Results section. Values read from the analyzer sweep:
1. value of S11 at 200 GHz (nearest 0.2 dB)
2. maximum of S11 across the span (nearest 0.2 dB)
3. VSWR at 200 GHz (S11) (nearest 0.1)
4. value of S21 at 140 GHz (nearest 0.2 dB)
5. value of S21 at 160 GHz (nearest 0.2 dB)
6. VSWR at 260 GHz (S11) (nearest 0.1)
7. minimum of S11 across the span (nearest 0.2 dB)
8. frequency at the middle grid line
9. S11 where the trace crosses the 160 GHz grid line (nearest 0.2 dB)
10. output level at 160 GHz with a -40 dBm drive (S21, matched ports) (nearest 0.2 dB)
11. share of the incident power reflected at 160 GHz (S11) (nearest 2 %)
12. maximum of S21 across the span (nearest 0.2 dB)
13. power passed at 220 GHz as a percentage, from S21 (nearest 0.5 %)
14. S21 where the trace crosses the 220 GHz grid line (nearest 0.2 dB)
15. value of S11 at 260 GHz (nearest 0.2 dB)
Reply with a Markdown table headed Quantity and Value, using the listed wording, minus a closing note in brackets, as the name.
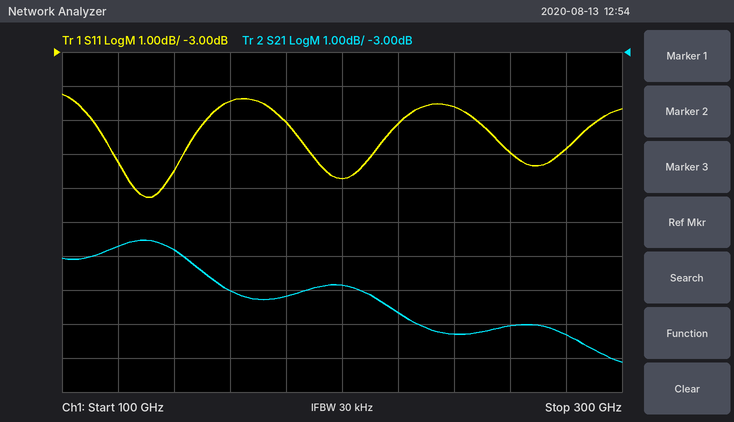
| Quantity | Value |
|---|---|
| value of S11 at 200 GHz | -6.8 dB |
| maximum of S11 across the span | -4.2 dB |
| VSWR at 200 GHz (S11) | 2.7 |
| value of S21 at 140 GHz | -8.8 dB |
| value of S21 at 160 GHz | -10.0 dB |
| VSWR at 260 GHz (S11) | 3.0 |
| minimum of S11 across the span | -7.2 dB |
| frequency at the middle grid line | 200 GHz |
| S11 where the trace crosses the 160 GHz grid line | -4.4 dB |
| output level at 160 GHz with a -40 dBm drive (S21, matched ports) | -50.0 dBm |
| share of the incident power reflected at 160 GHz (S11) | 36 % |
| maximum of S21 across the span | -8.6 dB |
| power passed at 220 GHz as a percentage, from S21 | 8.5 % |
| S21 where the trace crosses the 220 GHz grid line | -10.6 dB |
| value of S11 at 260 GHz | -6.0 dB |
